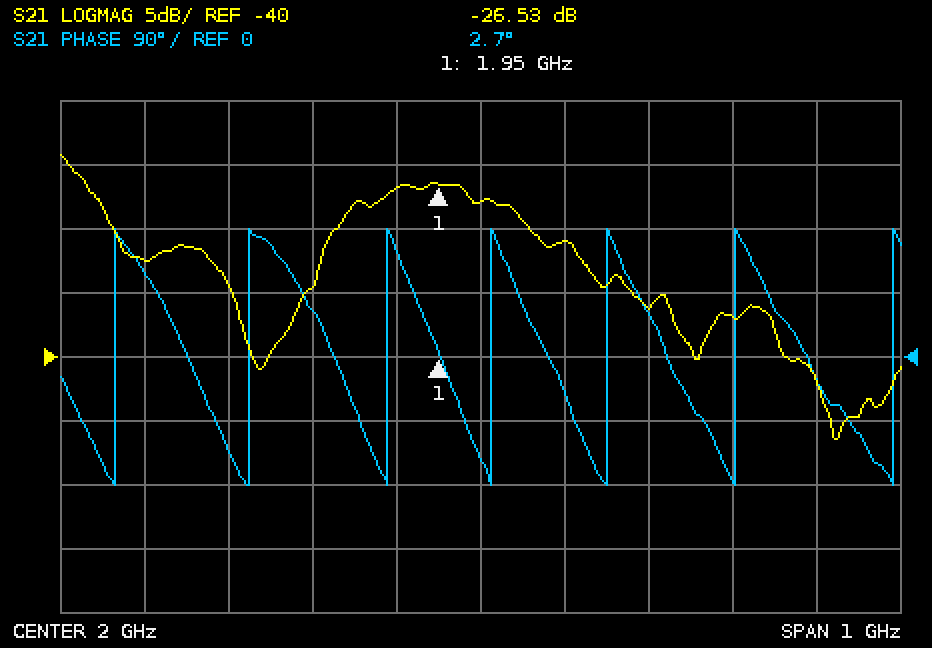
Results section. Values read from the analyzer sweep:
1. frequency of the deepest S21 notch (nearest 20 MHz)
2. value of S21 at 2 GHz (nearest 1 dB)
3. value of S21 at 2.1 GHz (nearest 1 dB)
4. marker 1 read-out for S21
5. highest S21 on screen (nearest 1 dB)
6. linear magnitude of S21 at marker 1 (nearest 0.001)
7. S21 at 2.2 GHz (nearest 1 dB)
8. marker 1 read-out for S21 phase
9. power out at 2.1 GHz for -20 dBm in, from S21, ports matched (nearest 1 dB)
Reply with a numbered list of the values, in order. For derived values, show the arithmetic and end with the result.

1. 2.42 GHz
2. -28 dB
3. -31 dB
4. -26.53 dB
5. -24 dB
6. 10^(-26.53/20) ≈ 0.047
7. -36 dB
8. 2.7°
9. -20 dBm + (-31 dB) = -51 dBm
